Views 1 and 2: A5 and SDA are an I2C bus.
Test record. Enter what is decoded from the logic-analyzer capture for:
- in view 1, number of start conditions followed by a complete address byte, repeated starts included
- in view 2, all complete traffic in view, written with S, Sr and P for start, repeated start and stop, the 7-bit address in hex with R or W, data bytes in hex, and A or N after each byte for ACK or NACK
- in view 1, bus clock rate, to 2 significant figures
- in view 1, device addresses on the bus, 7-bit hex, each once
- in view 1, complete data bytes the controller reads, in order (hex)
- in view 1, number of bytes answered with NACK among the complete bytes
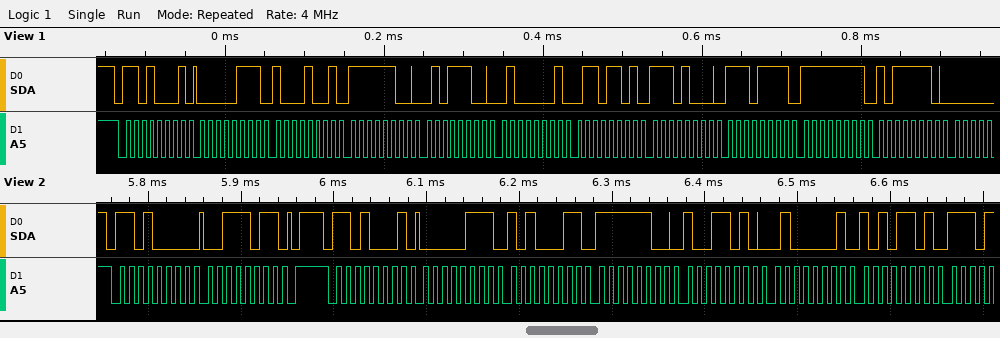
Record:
1
S 68W A 3B A P S 68R A 07 A A3 A FC A 9A A 41 A AD A
100 kHz
0x68
07 89 FC 5C 41 6D E8 EF FF BE
0
